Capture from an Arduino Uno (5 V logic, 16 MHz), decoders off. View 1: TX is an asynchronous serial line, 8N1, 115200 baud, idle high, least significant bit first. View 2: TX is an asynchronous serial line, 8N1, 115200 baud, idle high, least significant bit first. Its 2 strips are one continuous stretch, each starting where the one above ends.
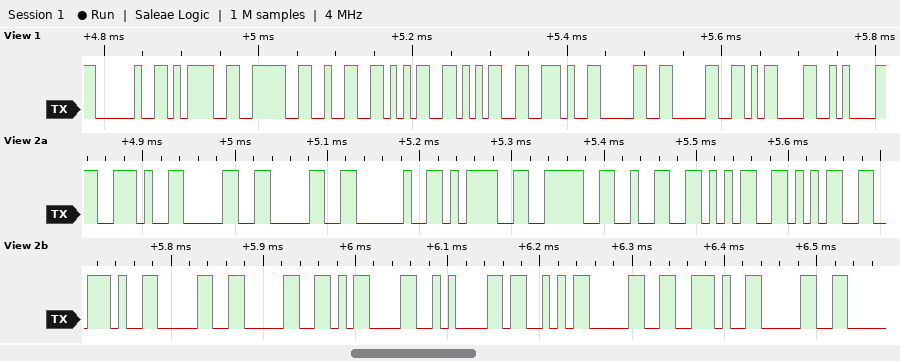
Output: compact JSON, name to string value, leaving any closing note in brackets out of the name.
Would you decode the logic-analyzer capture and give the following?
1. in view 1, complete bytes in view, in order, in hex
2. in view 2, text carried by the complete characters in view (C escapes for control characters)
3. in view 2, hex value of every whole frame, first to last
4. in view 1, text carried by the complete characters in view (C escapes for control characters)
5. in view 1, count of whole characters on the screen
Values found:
{"in view 1, complete bytes in view, in order, in hex": "20 3D 3E 32 35 35 2E 30 30 0D 0A", "in view 2, text carried by the complete characters in view": "\".00 =>255.00\\r\\nS0.0\"", "in view 2, hex value of every whole frame, first to last": "2E 30 30 20 3D 3E 32 35 35 2E 30 30 0D 0A 53 30 2E 30", "in view 1, text carried by the complete characters in view": "\" =>255.00\\r\\n\"", "in view 1, count of whole characters on the screen": "11"}
